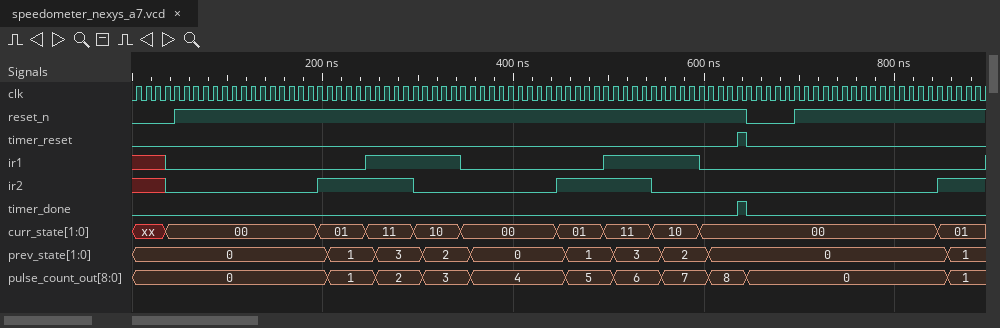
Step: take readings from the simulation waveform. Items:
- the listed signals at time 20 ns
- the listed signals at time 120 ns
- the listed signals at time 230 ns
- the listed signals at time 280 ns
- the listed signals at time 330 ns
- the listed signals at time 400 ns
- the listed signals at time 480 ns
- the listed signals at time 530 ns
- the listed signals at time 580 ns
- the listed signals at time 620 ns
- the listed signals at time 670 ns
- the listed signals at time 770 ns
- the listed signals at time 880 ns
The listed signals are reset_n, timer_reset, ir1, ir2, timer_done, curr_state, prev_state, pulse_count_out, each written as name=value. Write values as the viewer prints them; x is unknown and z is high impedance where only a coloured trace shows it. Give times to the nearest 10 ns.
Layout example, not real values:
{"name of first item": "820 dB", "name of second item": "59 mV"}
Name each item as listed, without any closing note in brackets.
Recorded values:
{"the listed signals at time 20 ns": "reset_n=0, timer_reset=0, ir1=x, ir2=x, timer_done=0, curr_state=xx, prev_state=0, pulse_count_out=0", "the listed signals at time 120 ns": "reset_n=1, timer_reset=0, ir1=0, ir2=0, timer_done=0, curr_state=00, prev_state=0, pulse_count_out=0", "the listed signals at time 230 ns": "reset_n=1, timer_reset=0, ir1=0, ir2=1, timer_done=0, curr_state=01, prev_state=1, pulse_count_out=1", "the listed signals at time 280 ns": "reset_n=1, timer_reset=0, ir1=1, ir2=1, timer_done=0, curr_state=11, prev_state=3, pulse_count_out=2", "the listed signals at time 330 ns": "reset_n=1, timer_reset=0, ir1=1, ir2=0, timer_done=0, curr_state=10, prev_state=2, pulse_count_out=3", "the listed signals at time 400 ns": "reset_n=1, timer_reset=0, ir1=0, ir2=0, timer_done=0, curr_state=00, prev_state=0, pulse_count_out=4", "the listed signals at time 480 ns": "reset_n=1, timer_reset=0, ir1=0, ir2=1, timer_done=0, curr_state=01, prev_state=1, pulse_count_out=5", "the listed signals at time 530 ns": "reset_n=1, timer_reset=0, ir1=1, ir2=1, timer_done=0, curr_state=11, prev_state=3, pulse_count_out=6", "the listed signals at time 580 ns": "reset_n=1, timer_reset=0, ir1=1, ir2=0, timer_done=0, curr_state=10, prev_state=2, pulse_count_out=7", "the listed signals at time 620 ns": "reset_n=1, timer_reset=0, ir1=0, ir2=0, timer_done=0, curr_state=00, prev_state=0, pulse_count_out=8", "the listed signals at time 670 ns": "reset_n=0, timer_reset=0, ir1=0, ir2=0, timer_done=0, curr_state=00, prev_state=0, pulse_count_out=0", "the listed signals at time 770 ns": "reset_n=1, timer_reset=0, ir1=0, ir2=0, timer_done=0, curr_state=00, prev_state=0, pulse_count_out=0", "the listed signals at time 880 ns": "reset_n=1, timer_reset=0, ir1=0, ir2=1, timer_done=0, curr_state=01, prev_state=1, pulse_count_out=1"}
